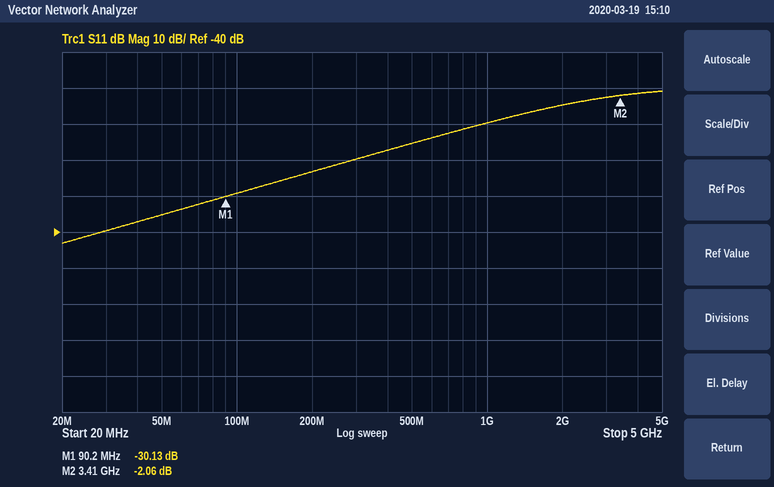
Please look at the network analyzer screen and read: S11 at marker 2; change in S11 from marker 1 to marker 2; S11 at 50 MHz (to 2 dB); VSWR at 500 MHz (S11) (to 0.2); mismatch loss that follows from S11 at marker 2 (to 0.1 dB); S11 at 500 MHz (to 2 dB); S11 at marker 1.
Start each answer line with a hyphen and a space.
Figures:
- -2.06 dB
- 28.07 dB
- -36 dB
- 1.4
- 4.2 dB
- -16 dB
- -30.13 dB
